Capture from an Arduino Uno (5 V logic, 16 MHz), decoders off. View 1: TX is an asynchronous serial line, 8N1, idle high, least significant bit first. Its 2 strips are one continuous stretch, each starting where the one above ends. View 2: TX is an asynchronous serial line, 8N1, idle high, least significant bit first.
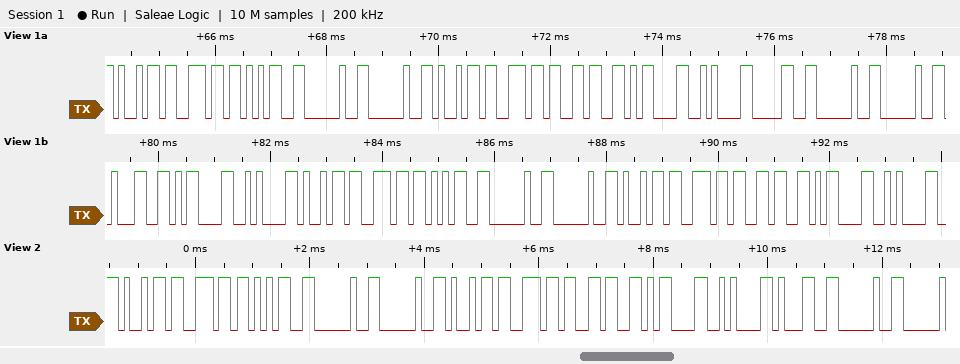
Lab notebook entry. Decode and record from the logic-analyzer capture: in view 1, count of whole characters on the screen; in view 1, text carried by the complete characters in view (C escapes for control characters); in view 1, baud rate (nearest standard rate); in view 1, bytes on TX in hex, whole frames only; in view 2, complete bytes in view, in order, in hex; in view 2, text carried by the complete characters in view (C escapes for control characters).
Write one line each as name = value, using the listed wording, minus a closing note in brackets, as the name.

in view 1, count of whole characters on the screen = 26
in view 1, text carried by the complete characters in view = "in5  in6\r\n0  1\r\nin5  in6\r\n"
in view 1, baud rate = 9600 baud
in view 1, bytes on TX in hex, whole frames only = 69 6E 35 20 20 69 6E 36 0D 0A 30 20 20 31 0D 0A 69 6E 35 20 20 69 6E 36 0D 0A
in view 2, complete bytes in view, in order, in hex = 69 6E 35 20 20 69 6E 36 0D 0A 31 20
in view 2, text carried by the complete characters in view = "in5  in6\r\n1 "
